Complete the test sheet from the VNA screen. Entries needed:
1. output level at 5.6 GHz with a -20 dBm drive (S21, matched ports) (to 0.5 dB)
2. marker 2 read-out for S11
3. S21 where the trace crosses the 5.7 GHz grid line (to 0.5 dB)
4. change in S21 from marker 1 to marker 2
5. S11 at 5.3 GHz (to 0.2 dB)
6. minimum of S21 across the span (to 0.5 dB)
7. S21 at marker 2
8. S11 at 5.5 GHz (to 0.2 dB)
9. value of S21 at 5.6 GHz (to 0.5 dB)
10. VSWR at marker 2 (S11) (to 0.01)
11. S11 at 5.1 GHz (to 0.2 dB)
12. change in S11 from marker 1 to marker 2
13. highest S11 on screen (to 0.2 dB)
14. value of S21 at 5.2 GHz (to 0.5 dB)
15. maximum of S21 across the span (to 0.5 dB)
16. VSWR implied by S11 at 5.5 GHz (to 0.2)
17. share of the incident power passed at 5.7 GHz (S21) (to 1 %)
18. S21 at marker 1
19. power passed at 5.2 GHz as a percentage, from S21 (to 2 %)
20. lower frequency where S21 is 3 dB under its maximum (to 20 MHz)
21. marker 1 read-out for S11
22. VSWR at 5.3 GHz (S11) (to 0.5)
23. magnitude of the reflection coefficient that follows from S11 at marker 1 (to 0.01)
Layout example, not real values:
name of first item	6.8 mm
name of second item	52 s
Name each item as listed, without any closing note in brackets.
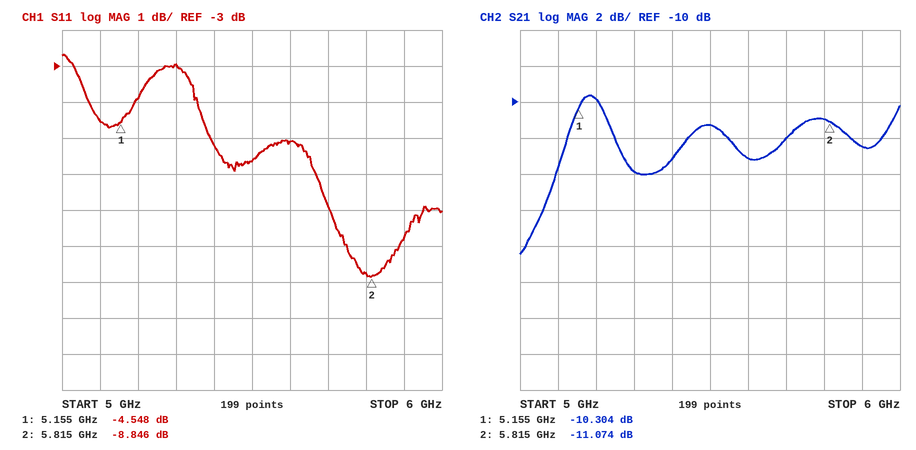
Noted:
output level at 5.6 GHz with a -20 dBm drive (S21, matched ports)	-33.0 dBm
marker 2 read-out for S11	-8.846 dB
S21 where the trace crosses the 5.7 GHz grid line	-12.0 dB
change in S21 from marker 1 to marker 2	-0.770 dB
S11 at 5.3 GHz	-3.0 dB
minimum of S21 across the span	-18.5 dB
S21 at marker 2	-11.074 dB
S11 at 5.5 GHz	-5.6 dB
value of S21 at 5.6 GHz	-13.0 dB
VSWR at marker 2 (S11)	2.13
S11 at 5.1 GHz	-4.6 dB
change in S11 from marker 1 to marker 2	-4.298 dB
highest S11 on screen	-2.6 dB
value of S21 at 5.2 GHz	-10.0 dB
maximum of S21 across the span	-9.5 dB
VSWR implied by S11 at 5.5 GHz	3.2
share of the incident power passed at 5.7 GHz (S21)	6 %
S21 at marker 1	-10.304 dB
power passed at 5.2 GHz as a percentage, from S21	10 %
lower frequency where S21 is 3 dB under its maximum	5.12 GHz
marker 1 read-out for S11	-4.548 dB
VSWR at 5.3 GHz (S11)	6.0
magnitude of the reflection coefficient that follows from S11 at marker 1	0.59
